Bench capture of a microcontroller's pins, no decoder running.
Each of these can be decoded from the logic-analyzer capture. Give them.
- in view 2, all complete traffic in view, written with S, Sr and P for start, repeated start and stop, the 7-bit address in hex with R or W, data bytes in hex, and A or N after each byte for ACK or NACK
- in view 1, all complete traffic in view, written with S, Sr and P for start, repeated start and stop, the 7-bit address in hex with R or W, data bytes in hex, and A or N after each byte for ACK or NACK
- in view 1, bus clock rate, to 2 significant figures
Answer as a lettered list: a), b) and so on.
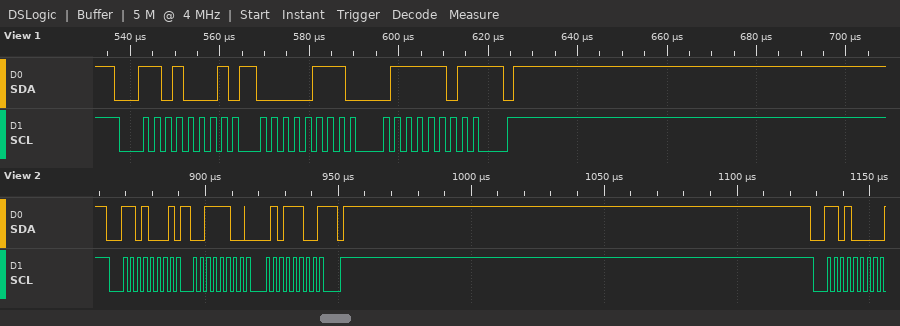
a) S 68R A 3C A 5C N P S 68W A
b) S 68R A 07 A 7D N P
c) 400 kHz
